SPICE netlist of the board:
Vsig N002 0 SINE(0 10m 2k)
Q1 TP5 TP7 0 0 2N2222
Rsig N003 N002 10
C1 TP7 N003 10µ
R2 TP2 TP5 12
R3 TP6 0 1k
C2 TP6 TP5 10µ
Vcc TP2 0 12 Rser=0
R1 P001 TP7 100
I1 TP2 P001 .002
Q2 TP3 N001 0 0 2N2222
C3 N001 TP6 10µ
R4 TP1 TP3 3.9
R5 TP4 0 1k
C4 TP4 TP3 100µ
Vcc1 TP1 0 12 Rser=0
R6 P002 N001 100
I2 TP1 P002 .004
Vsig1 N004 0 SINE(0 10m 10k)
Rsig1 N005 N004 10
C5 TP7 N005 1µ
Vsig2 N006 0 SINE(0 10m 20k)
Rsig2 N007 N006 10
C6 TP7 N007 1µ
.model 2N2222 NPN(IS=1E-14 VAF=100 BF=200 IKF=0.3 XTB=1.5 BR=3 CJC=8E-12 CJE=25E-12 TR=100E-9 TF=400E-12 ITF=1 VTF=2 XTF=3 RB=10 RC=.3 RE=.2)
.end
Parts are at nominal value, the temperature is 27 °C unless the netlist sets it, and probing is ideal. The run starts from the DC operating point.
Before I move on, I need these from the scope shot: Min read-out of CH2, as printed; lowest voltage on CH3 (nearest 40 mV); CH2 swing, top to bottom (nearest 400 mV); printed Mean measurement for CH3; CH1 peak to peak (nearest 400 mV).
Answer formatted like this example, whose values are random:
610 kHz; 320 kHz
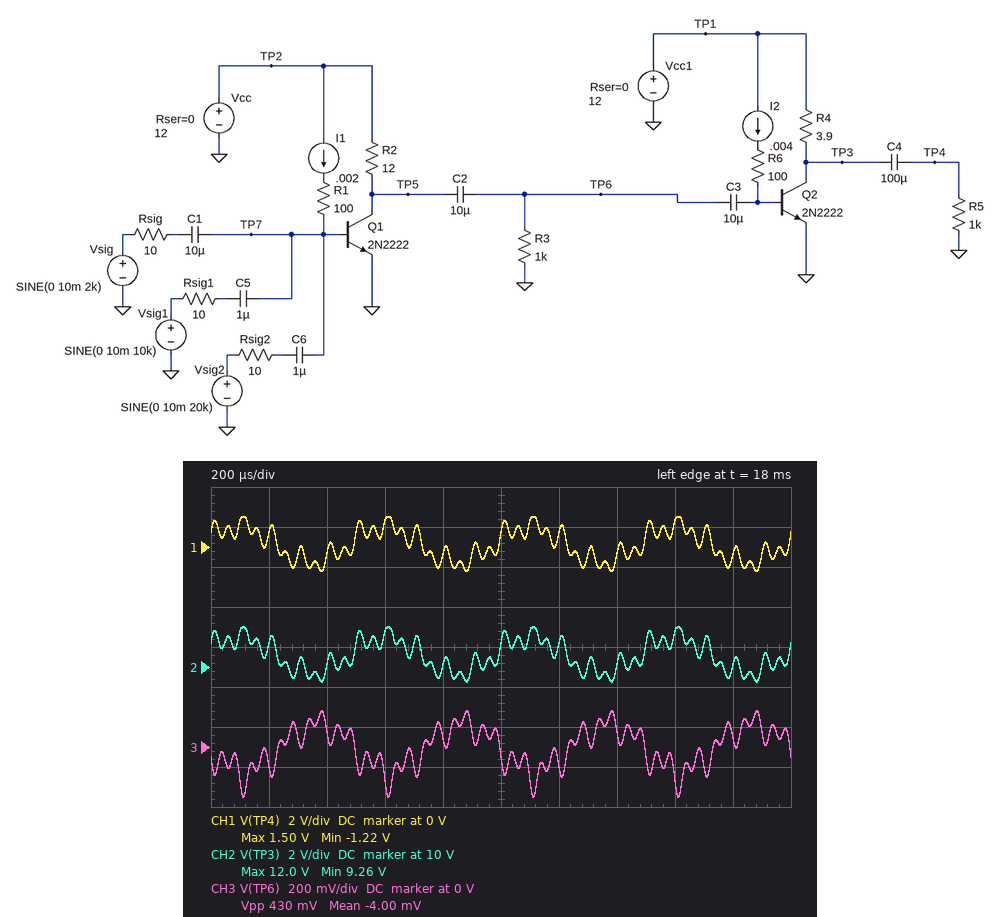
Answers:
9.26 V; -240 mV; 2.8 V; -4.00 mV; 2.8 V
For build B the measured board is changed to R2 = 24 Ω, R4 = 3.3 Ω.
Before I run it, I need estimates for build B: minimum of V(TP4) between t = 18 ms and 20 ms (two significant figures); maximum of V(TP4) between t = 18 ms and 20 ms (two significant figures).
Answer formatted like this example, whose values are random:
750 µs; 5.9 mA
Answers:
-1.4 V; 1.3 V
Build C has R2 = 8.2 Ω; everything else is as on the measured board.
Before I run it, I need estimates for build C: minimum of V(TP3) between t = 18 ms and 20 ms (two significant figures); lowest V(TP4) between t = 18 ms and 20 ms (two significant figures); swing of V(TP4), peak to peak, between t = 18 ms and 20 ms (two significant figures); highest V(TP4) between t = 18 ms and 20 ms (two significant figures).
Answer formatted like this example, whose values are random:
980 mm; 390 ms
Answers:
9.5 V; -960 mV; 2.3 V; 1.3 V
